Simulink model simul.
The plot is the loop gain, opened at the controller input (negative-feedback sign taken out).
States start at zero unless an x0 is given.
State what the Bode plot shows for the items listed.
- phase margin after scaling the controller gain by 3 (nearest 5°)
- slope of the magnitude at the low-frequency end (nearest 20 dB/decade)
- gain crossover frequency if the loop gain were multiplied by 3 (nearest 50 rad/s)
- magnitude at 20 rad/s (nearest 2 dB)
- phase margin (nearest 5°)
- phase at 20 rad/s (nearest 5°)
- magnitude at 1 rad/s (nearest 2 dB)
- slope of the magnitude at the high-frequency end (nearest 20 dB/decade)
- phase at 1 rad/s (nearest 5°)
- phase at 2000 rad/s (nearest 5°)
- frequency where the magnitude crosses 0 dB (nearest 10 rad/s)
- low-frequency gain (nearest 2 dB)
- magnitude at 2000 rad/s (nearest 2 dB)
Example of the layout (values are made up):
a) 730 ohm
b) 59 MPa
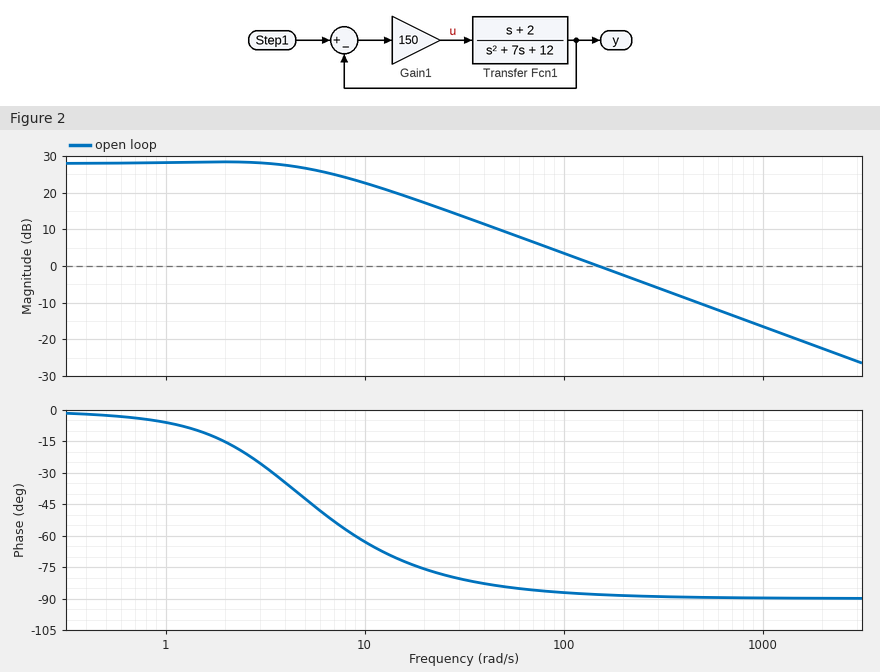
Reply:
a) 90°
b) 0 dB/decade
c) 450 rad/s
d) 18 dB
e) 90°
f) -75°
g) 28 dB
h) -20 dB/decade
i) -5°
j) -90°
k) 150 rad/s
l) 28 dB
m) -22 dB
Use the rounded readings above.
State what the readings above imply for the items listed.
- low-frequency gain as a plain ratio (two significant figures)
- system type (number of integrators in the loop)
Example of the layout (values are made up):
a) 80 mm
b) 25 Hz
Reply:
a) 25
b) 0
